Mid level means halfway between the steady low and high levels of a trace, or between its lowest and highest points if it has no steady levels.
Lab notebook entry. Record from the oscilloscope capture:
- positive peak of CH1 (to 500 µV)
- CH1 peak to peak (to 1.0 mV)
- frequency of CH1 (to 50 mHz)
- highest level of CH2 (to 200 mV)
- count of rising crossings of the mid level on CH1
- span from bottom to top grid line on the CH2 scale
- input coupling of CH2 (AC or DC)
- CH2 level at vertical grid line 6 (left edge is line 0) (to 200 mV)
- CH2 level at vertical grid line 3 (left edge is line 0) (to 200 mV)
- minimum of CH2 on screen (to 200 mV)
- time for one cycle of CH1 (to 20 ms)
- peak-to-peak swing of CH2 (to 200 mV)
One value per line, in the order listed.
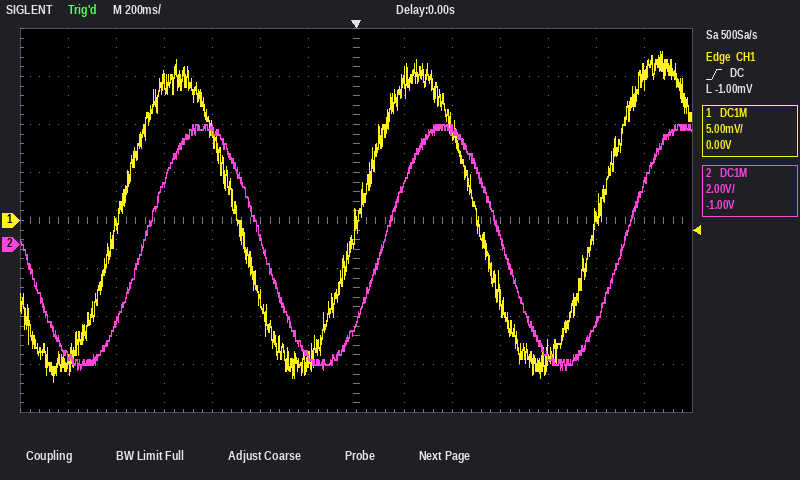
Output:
17.5 mV
34.0 mV
1.00 Hz
5.0 V
3
16 V
DC
-4.6 V
2.6 V
-5.2 V
1.00 s
10.2 V
